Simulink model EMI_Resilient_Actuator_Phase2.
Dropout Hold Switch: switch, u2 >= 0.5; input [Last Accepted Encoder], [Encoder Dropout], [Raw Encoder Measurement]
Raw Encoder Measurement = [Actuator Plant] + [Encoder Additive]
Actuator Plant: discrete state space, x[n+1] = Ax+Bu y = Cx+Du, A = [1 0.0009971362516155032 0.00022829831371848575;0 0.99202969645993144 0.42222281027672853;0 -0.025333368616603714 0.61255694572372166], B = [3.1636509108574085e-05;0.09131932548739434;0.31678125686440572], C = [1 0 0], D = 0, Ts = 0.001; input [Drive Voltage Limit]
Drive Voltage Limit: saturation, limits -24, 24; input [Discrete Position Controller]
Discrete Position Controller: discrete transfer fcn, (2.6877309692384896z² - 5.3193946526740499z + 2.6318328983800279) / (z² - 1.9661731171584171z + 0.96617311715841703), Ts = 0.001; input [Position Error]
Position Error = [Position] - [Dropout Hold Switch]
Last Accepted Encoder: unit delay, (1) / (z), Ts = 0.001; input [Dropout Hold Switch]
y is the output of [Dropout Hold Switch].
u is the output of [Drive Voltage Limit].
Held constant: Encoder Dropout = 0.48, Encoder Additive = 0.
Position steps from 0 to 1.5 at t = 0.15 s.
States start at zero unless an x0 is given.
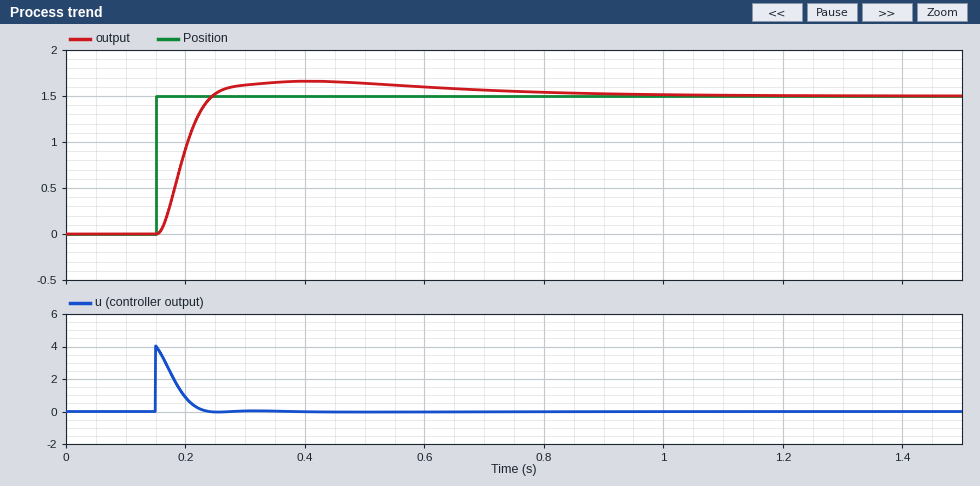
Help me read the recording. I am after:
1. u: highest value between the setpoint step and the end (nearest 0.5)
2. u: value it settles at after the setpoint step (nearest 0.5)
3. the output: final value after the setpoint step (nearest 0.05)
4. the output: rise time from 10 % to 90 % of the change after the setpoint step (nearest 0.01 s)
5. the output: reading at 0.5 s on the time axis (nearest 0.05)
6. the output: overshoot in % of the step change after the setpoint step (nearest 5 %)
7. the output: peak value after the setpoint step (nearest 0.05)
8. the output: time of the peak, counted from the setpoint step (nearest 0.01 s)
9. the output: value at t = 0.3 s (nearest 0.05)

4.0
0.0
1.50
0.06 s
1.65
10 %
1.65
0.26 s
1.60
